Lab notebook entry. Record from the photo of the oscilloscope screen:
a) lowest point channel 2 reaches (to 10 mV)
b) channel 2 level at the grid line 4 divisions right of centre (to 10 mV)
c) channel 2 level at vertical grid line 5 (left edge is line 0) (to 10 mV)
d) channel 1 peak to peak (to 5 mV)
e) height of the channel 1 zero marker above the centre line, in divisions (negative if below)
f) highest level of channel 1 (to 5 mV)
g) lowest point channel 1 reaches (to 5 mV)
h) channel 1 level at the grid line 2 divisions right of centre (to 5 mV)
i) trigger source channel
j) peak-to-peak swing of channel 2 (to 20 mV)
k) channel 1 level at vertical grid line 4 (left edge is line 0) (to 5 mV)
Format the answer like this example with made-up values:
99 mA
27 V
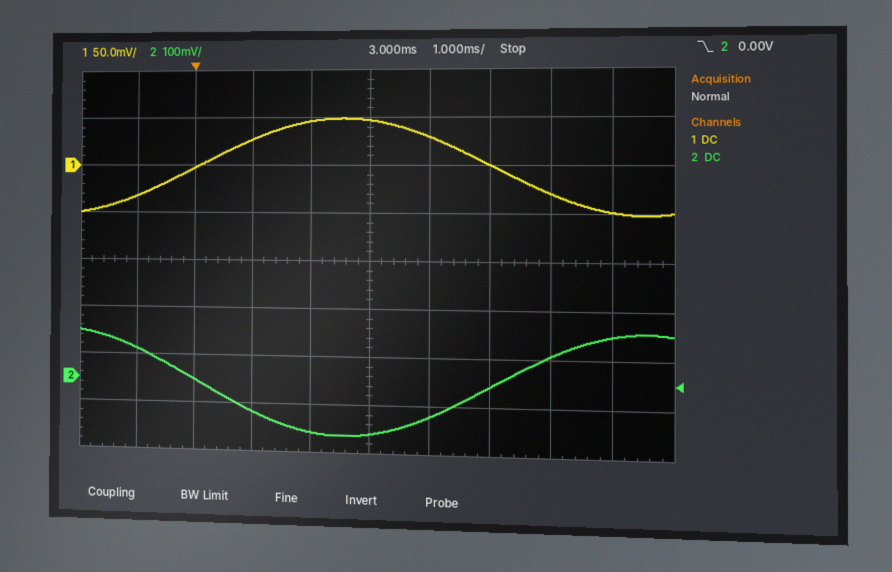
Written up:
-110 mV
100 mV
-110 mV
100 mV
+2.0 div
50 mV
-50 mV
0 mV
channel 2
220 mV
45 mV
